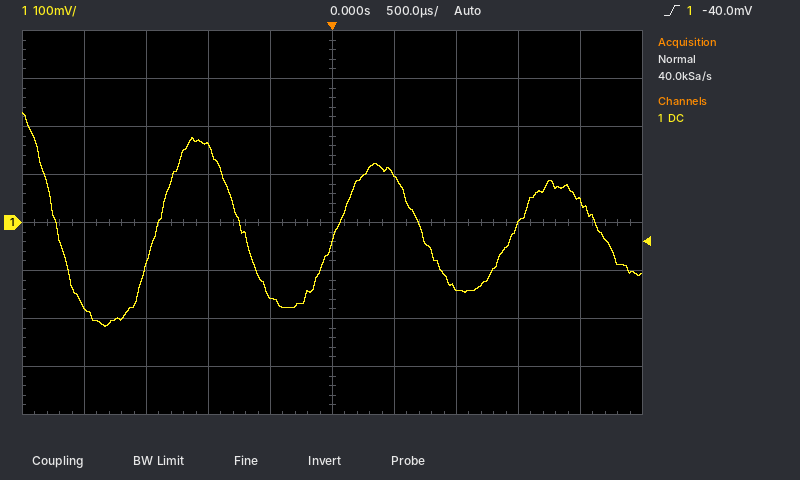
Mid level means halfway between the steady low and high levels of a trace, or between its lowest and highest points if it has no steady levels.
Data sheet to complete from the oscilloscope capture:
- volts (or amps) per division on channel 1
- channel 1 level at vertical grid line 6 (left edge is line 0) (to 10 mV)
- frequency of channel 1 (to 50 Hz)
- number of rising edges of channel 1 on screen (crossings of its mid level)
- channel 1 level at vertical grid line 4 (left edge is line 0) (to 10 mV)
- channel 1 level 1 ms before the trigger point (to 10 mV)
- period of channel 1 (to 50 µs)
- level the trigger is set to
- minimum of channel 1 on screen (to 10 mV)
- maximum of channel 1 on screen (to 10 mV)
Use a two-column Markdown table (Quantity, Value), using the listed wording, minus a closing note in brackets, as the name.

| Quantity | Value |
|---|---|
| volts (or amps) per division on channel 1 | 100 mV |
| channel 1 level at vertical grid line 6 (left edge is line 0) | 100 mV |
| frequency of channel 1 | 700 Hz |
| number of rising edges of channel 1 on screen | 3 |
| channel 1 level at vertical grid line 4 (left edge is line 0) | -150 mV |
| channel 1 level 1 ms before the trigger point | 160 mV |
| period of channel 1 | 1.45 ms |
| level the trigger is set to | -40.0 mV |
| minimum of channel 1 on screen | -220 mV |
| maximum of channel 1 on screen | 230 mV |
